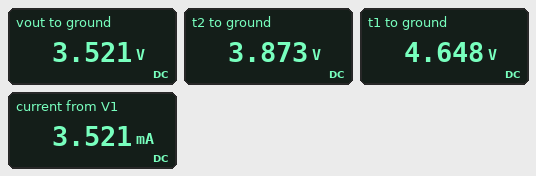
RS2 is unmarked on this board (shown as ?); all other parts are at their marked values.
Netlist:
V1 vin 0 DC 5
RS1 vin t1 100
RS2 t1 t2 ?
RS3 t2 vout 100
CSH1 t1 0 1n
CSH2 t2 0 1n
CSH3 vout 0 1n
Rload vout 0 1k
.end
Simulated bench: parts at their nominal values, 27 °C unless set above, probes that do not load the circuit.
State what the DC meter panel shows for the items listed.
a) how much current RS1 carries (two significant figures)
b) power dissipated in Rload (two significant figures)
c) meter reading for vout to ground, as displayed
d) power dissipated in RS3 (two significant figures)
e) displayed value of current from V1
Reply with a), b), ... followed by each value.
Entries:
a) 3.5 mA
b) 12 mW
c) 3.521 V
d) 1.2 mW
e) 3.521 mA
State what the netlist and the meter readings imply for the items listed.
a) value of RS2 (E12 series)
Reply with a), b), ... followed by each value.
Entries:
a) 220 Ω
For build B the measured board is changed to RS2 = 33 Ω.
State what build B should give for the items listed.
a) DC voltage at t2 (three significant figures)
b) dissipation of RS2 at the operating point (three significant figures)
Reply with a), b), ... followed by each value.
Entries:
a) 4.46 V
b) 543 µW
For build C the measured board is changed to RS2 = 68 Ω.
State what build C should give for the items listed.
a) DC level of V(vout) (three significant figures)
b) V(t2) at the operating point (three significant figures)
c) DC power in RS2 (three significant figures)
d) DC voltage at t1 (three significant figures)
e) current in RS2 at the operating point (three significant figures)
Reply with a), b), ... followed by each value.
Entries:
a) 3.94 V
b) 4.34 V
c) 1.06 mW
d) 4.61 V
e) 3.94 mA
